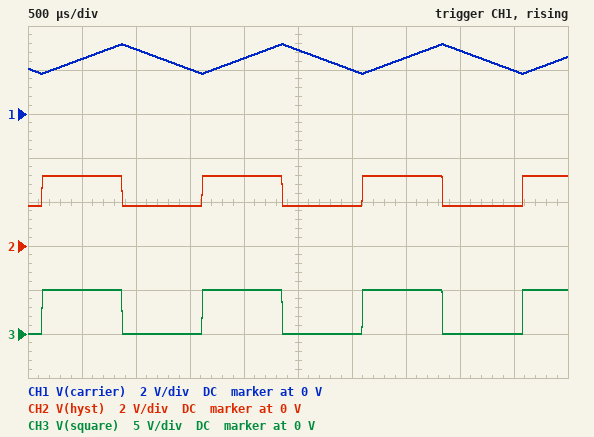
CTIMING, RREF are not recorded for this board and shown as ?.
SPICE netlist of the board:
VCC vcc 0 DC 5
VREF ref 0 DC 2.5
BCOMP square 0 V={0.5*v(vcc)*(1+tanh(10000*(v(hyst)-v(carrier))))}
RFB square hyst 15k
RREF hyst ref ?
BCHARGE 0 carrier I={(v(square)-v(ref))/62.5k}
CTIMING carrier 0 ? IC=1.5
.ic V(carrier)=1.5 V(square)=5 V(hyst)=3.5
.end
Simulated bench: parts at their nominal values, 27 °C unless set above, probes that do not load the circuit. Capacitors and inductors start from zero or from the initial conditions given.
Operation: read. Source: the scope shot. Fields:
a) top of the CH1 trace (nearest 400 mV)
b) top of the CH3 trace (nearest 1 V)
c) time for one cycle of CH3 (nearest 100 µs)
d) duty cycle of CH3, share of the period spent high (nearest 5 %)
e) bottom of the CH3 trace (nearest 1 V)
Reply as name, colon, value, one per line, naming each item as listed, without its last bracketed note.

top of the CH1 trace: 3.2 V
top of the CH3 trace: 5 V
time for one cycle of CH3: 1.5 ms
duty cycle of CH3, share of the period spent high: 50 %
bottom of the CH3 trace: 0 V
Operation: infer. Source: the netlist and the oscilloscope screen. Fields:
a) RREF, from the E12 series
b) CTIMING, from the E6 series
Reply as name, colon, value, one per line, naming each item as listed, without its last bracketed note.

RREF, from the E12 series: 5.6 kΩ
CTIMING, from the E6 series: 22 nF
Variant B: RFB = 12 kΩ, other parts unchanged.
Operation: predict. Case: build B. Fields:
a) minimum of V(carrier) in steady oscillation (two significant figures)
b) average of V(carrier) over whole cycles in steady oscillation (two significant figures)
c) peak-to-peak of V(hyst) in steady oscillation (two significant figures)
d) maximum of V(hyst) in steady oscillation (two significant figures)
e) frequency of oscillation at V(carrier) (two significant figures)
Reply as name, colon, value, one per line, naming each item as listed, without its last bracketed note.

minimum of V(carrier) in steady oscillation: 1.7 V
average of V(carrier) over whole cycles in steady oscillation: 2.5 V
peak-to-peak of V(hyst) in steady oscillation: 1.6 V
maximum of V(hyst) in steady oscillation: 3.3 V
frequency of oscillation at V(carrier): 570 Hz
